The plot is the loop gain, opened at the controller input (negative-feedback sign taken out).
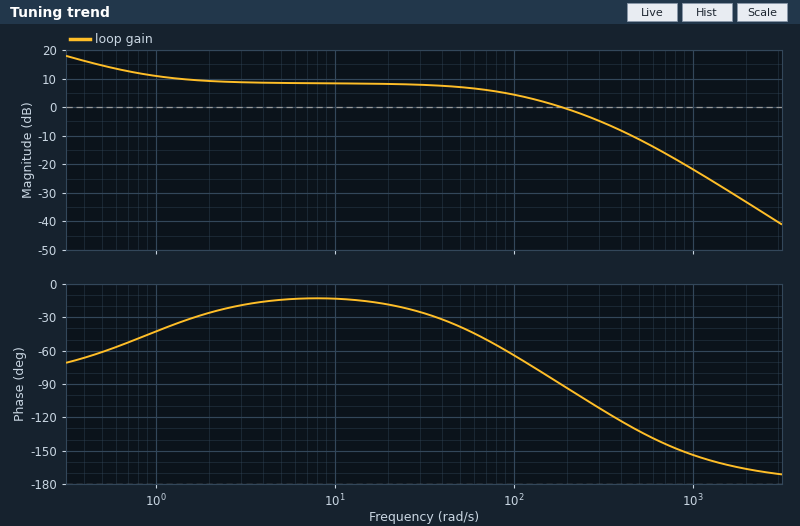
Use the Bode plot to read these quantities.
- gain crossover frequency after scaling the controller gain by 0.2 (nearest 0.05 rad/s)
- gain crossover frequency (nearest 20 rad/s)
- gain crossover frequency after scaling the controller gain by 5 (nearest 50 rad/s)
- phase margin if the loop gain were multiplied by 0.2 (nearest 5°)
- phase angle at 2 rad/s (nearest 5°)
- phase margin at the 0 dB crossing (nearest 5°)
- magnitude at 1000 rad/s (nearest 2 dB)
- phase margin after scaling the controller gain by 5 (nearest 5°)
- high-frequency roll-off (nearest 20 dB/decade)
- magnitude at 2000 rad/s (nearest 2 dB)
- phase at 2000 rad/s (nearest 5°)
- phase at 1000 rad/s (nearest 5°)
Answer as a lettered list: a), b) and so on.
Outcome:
a) 0.55 rad/s
b) 180 rad/s
c) 600 rad/s
d) 120°
e) -25°
f) 90°
g) -22 dB
h) 40°
i) -40 dB/decade
j) -34 dB
k) -165°
l) -155°
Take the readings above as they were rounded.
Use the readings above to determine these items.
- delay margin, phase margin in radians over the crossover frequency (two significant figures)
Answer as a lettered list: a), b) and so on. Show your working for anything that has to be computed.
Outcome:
a) 90 × π / 180 / 180 = 0.0087 s
